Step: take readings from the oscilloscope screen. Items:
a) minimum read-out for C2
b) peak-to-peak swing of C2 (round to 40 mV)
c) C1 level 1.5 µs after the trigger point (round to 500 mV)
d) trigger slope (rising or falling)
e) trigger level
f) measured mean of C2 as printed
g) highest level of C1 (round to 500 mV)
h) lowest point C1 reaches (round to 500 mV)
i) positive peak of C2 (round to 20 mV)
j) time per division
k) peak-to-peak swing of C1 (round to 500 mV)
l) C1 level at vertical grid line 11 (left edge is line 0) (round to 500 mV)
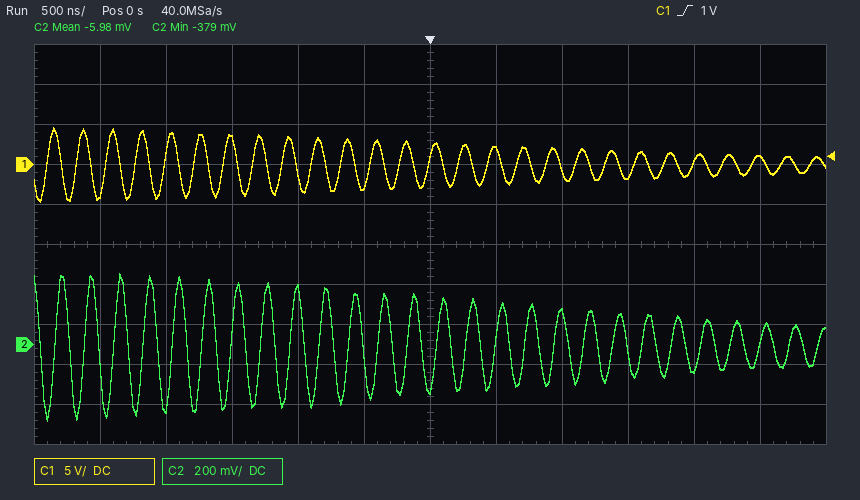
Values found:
-379 mV
720 mV
-1.5 V
rising
1 V
-5.98 mV
4.5 V
-4.5 V
360 mV
500 ns
9.0 V
1.0 V
